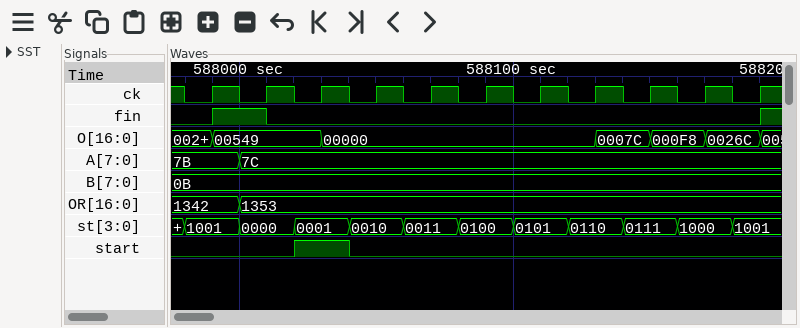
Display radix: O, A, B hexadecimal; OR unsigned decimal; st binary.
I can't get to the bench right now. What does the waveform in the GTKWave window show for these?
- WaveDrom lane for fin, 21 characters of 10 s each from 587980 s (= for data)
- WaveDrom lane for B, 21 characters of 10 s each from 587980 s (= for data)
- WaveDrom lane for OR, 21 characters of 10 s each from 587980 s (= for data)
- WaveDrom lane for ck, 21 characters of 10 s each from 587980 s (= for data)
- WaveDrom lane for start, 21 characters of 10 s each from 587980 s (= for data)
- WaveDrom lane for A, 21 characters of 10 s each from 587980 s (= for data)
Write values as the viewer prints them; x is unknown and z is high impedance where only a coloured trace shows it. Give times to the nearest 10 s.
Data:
{name: 'fin', wave: '01.0.................'}
{name: 'B', wave: '=....................', data: '0B'}
{name: 'OR', wave: '=.=..................', data: '1342 1353'}
{name: 'ck', wave: '010101010101010101010'}
{name: 'start', wave: '0...1.0..............'}
{name: 'A', wave: '=.=..................', data: '7B 7C'}
